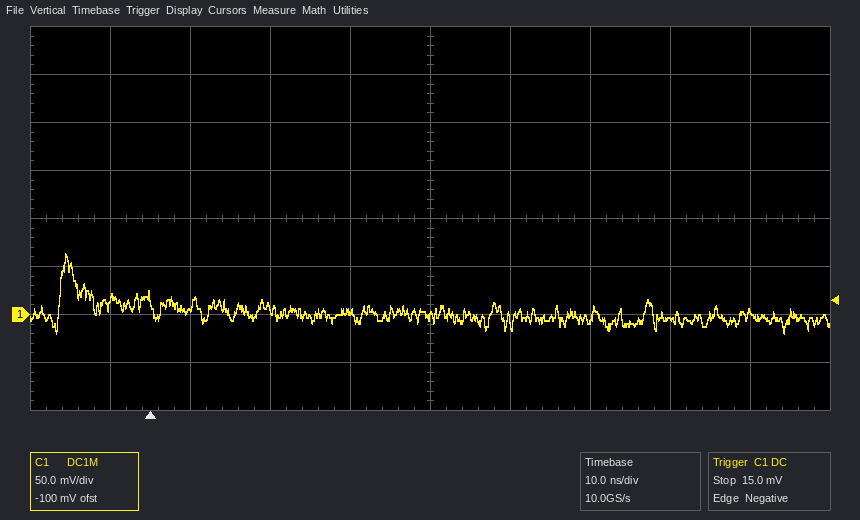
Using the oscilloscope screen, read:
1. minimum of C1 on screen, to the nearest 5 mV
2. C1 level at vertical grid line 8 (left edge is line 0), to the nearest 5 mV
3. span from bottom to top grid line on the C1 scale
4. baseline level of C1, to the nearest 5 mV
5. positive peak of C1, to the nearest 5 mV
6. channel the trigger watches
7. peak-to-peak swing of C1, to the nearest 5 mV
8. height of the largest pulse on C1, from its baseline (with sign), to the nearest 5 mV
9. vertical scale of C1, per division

-20 mV
-5 mV
400 mV
0 mV
65 mV
C1
85 mV
+65 mV
50 mV
